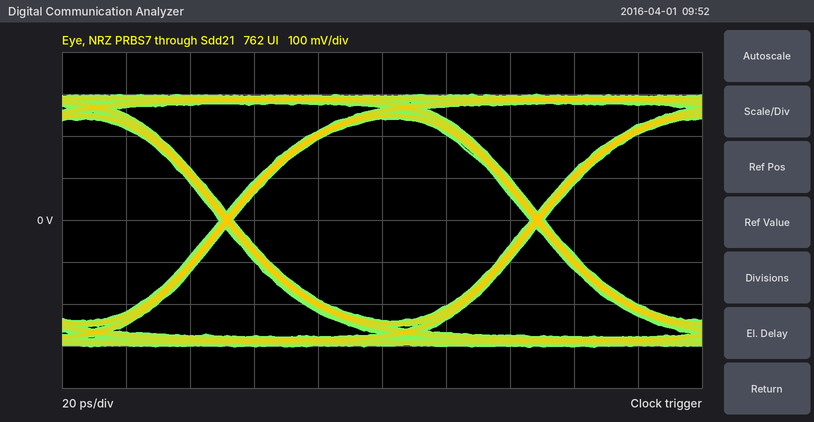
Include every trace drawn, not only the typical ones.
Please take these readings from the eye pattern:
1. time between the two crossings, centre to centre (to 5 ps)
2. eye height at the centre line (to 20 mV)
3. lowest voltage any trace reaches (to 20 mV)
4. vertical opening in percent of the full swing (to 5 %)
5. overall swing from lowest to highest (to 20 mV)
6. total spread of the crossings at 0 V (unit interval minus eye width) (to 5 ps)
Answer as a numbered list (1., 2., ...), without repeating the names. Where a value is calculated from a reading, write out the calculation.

1. 95 ps
2. 480 mV
3. -300 mV
4. 480 mV / 600 mV ≈ 80 %
5. 600 mV
6. 5 ps
